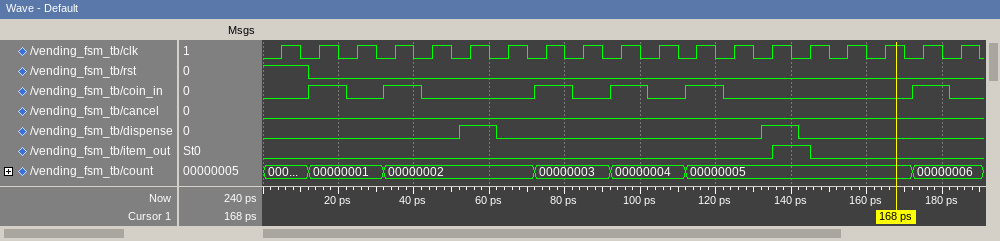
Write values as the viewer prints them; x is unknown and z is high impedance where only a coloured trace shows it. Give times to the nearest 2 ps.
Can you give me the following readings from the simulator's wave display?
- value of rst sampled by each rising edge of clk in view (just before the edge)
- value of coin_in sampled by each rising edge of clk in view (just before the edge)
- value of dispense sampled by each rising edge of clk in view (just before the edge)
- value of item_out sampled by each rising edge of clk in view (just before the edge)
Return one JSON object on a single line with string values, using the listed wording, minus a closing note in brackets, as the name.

{"value of rst sampled by each rising edge of clk in view": "1 0 0 0 0 0 0 0 0 0 0 0 0 0 0 0 0 0 0", "value of coin_in sampled by each rising edge of clk in view": "0 1 0 1 0 0 0 1 0 1 0 1 0 0 0 0 0 1 0", "value of dispense sampled by each rising edge of clk in view": "0 0 0 0 0 1 0 0 0 0 0 0 0 1 0 0 0 0 0", "value of item_out sampled by each rising edge of clk in view": "0 0 0 0 0 0 0 0 0 0 0 0 0 0 1 0 0 0 0"}
